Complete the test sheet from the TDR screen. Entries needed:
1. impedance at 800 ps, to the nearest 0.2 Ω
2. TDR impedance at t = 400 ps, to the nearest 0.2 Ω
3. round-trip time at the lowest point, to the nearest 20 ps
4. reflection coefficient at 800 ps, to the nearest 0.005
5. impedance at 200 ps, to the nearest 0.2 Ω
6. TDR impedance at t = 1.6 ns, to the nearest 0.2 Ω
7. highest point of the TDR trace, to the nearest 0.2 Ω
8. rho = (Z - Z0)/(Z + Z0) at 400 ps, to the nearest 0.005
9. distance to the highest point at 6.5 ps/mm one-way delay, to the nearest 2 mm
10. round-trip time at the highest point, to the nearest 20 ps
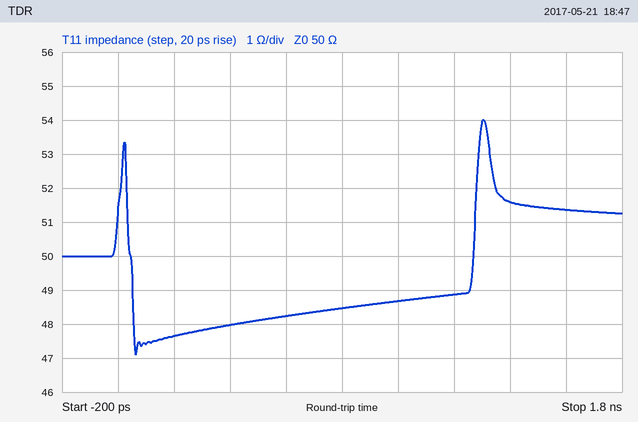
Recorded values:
48.4 Ω
48.0 Ω
60 ps
-0.015
47.6 Ω
51.4 Ω
54.0 Ω
-0.020
100 mm
1.30 ns
